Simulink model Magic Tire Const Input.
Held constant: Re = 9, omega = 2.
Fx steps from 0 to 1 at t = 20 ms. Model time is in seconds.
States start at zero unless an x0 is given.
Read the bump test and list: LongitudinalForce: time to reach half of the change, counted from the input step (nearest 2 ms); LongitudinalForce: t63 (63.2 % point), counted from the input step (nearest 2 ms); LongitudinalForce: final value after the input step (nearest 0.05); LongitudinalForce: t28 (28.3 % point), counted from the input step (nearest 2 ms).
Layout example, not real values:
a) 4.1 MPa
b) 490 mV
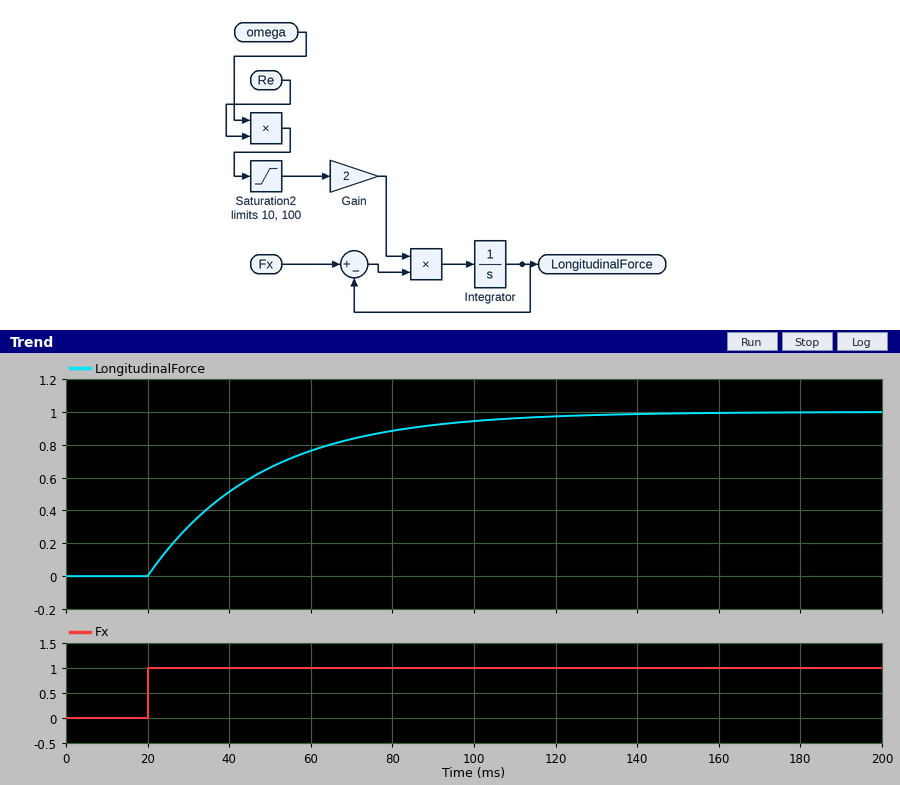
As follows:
a) 20 ms
b) 28 ms
c) 1.00
d) 10 ms
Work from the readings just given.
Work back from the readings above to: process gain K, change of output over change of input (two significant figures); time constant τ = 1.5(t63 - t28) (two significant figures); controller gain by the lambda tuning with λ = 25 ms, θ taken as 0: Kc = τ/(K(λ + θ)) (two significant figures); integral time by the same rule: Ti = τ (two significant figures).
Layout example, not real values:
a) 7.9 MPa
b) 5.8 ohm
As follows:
a) 1.0
b) 27 ms
c) 1.1
d) 27 ms
